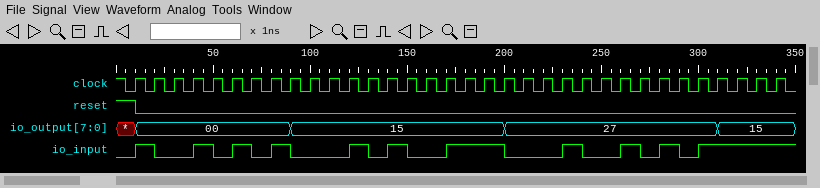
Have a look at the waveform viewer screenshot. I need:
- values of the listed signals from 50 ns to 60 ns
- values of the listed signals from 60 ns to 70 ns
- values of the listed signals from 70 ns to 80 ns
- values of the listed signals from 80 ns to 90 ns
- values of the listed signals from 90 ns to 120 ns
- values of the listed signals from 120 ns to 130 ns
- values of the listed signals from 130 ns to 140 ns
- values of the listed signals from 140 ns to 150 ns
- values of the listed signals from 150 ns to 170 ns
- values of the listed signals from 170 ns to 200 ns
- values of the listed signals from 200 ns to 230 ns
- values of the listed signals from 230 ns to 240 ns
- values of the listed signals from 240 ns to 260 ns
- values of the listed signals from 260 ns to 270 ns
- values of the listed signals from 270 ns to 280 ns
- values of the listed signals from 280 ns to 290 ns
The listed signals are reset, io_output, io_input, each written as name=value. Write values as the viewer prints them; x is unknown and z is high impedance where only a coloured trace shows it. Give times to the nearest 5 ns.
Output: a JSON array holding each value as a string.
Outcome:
["reset=0, io_output=00, io_input=0", "reset=0, io_output=00, io_input=1", "reset=0, io_output=00, io_input=0", "reset=0, io_output=00, io_input=1", "reset=0, io_output=15, io_input=0", "reset=0, io_output=15, io_input=1", "reset=0, io_output=15, io_input=0", "reset=0, io_output=15, io_input=1", "reset=0, io_output=15, io_input=0", "reset=0, io_output=15, io_input=1", "reset=0, io_output=27, io_input=0", "reset=0, io_output=27, io_input=1", "reset=0, io_output=27, io_input=0", "reset=0, io_output=27, io_input=1", "reset=0, io_output=27, io_input=0", "reset=0, io_output=27, io_input=1"]
